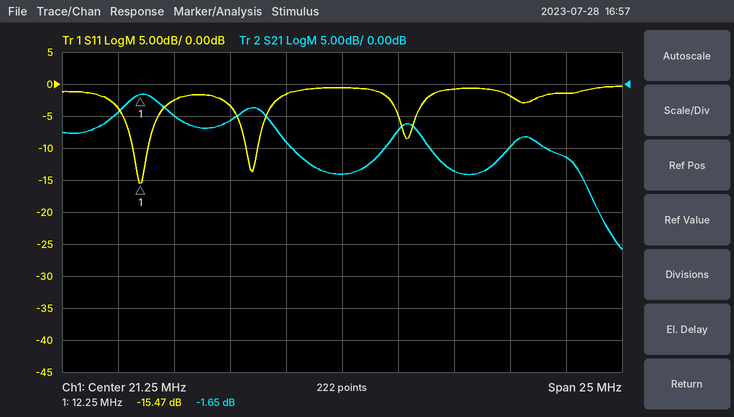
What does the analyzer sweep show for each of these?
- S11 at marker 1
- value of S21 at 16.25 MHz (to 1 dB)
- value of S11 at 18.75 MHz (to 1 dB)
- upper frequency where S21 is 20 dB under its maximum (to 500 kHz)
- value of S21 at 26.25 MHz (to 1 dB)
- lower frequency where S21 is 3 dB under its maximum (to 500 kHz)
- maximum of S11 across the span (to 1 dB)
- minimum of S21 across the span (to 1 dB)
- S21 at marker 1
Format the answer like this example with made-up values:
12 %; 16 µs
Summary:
-15.47 dB; -6 dB; -2 dB; 33.0 MHz; -14 dB; 11.0 MHz; 0 dB; -26 dB; -1.65 dB
